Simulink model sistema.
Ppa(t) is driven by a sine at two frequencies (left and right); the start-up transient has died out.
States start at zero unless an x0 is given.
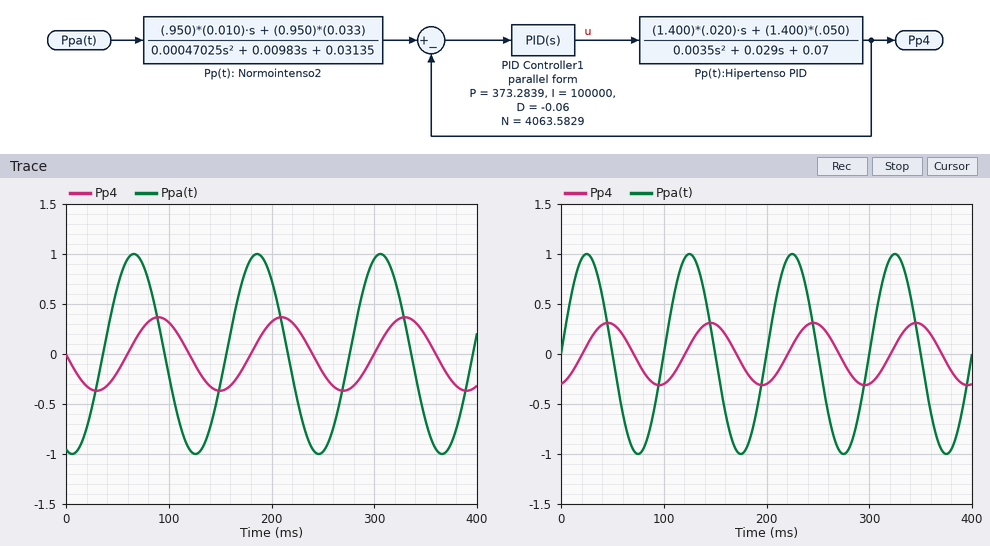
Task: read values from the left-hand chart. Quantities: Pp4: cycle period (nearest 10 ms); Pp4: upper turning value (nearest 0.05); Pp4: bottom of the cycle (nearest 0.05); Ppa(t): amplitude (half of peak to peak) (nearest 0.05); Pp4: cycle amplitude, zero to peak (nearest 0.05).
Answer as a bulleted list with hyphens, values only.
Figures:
- 120 ms
- 0.35
- -0.35
- 1.00
- 0.35
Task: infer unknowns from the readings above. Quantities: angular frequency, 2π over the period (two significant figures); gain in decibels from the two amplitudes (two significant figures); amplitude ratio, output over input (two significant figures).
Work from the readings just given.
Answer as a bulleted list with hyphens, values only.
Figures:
- 0.052 rad/ms
- -9.1 dB
- 0.35
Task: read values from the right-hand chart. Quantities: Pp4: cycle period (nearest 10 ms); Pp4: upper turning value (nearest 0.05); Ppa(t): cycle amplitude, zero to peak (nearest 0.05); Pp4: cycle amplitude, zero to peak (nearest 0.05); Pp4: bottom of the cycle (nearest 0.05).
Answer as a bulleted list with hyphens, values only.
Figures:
- 100 ms
- 0.30
- 1.00
- 0.30
- -0.30
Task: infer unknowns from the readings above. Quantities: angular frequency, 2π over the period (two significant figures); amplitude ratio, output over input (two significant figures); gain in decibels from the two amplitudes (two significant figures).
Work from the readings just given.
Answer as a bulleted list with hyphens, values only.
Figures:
- 0.063 rad/ms
- 0.30
- -10 dB
